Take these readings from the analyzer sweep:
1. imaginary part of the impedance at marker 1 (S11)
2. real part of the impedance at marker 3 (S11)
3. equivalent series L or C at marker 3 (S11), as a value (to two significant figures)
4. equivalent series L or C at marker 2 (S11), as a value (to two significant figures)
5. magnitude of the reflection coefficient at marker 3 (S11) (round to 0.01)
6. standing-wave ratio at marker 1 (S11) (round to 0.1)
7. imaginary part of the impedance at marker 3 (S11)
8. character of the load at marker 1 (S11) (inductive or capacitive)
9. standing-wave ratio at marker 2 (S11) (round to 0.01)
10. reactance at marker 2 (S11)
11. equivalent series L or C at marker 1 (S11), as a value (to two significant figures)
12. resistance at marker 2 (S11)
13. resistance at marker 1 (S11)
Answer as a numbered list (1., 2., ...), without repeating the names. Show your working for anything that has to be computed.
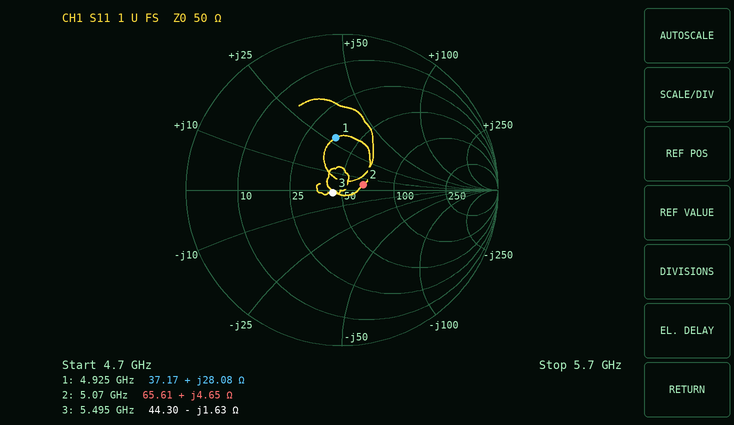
1. +28.08 Ω
2. 44.30 Ω
3. C = 1/(2π × 5.495 GHz × 1.63 Ω) ≈ 18 pF
4. L = 4.65 Ω/(2π × 5.07 GHz) ≈ 146 pH, so 150 pH to two significant figures
5. 0.06
6. 2.0
7. -1.63 Ω
8. inductive
9. 1.33
10. +4.65 Ω
11. L = 28.08 Ω/(2π × 4.925 GHz) ≈ 907 pH, so 910 pH to two significant figures
12. 65.61 Ω
13. 37.17 Ω
